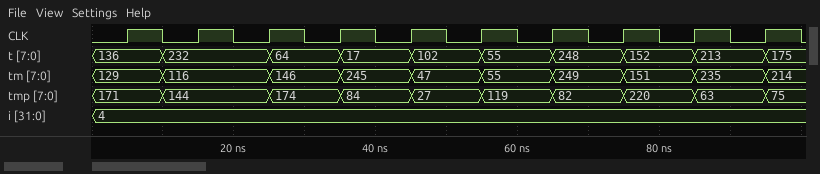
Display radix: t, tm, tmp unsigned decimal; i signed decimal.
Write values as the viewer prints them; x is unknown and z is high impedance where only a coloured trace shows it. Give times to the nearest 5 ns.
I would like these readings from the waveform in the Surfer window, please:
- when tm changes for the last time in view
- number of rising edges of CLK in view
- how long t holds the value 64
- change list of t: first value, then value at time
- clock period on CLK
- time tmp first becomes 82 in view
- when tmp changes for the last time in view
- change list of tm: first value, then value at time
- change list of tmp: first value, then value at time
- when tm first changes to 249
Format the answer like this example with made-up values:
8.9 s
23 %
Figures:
95 ns
10
10 ns
136, 232 at 10 ns, 64 at 25 ns, 17 at 35 ns, 102 at 45 ns, 55 at 55 ns, 248 at 65 ns, 152 at 75 ns, 213 at 85 ns, 175 at 95 ns
10 ns
65 ns
95 ns
129, 116 at 10 ns, 146 at 25 ns, 245 at 35 ns, 47 at 45 ns, 55 at 55 ns, 249 at 65 ns, 151 at 75 ns, 235 at 85 ns, 214 at 95 ns
171, 144 at 10 ns, 174 at 25 ns, 84 at 35 ns, 27 at 45 ns, 119 at 55 ns, 82 at 65 ns, 220 at 75 ns, 63 at 85 ns, 75 at 95 ns
65 ns
